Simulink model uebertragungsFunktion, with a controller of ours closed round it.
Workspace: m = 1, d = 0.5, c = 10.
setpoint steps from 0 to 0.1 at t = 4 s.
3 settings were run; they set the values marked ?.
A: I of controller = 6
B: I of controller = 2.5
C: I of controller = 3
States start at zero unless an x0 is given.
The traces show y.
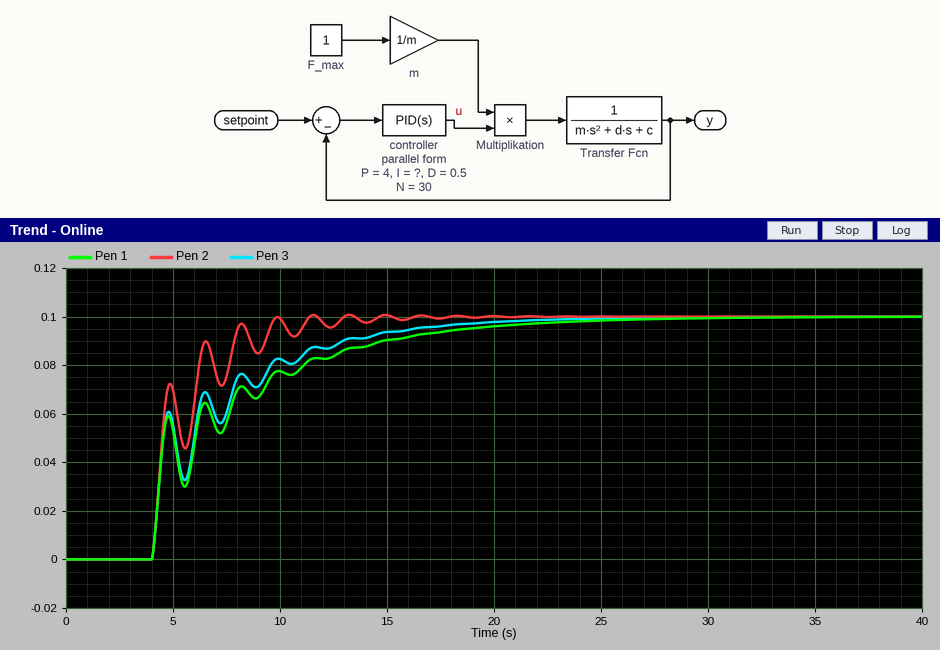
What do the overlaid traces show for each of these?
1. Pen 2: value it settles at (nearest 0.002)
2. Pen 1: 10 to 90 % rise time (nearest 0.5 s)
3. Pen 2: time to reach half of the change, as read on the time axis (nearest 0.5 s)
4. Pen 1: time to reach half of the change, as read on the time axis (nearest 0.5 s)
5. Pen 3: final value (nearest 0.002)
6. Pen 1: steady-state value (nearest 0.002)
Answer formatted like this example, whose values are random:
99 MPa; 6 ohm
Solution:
0.100; 10.5 s; 4.5 s; 4.5 s; 0.100; 0.100
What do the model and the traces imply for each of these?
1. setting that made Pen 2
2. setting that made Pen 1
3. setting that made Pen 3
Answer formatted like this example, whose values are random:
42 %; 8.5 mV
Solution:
A; B; C
